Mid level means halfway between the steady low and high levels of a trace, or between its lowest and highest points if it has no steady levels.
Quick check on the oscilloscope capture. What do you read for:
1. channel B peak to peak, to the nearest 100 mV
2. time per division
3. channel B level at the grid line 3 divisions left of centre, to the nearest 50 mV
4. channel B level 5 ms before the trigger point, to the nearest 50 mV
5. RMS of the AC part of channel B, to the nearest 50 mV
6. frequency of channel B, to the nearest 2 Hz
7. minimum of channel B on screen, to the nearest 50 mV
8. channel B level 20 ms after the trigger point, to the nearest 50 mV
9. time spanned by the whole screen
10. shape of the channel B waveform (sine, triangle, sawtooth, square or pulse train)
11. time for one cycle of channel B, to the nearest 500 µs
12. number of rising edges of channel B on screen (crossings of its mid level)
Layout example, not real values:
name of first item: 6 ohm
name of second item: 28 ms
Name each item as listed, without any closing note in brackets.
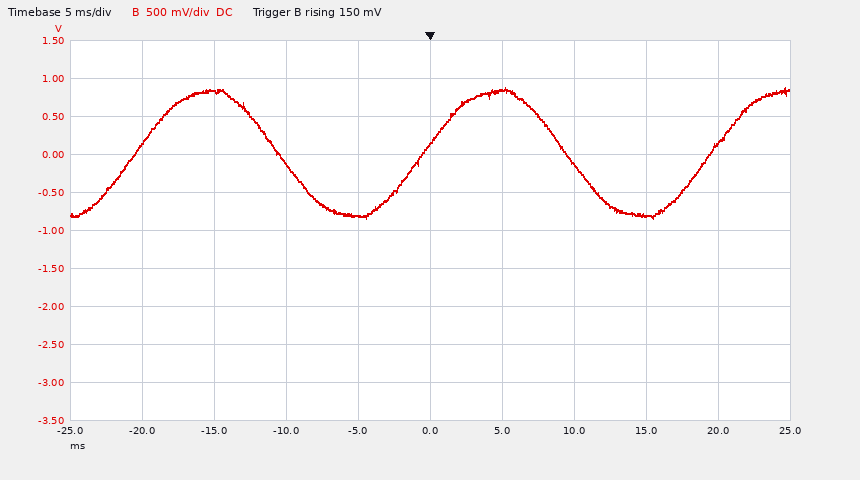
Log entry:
channel B peak to peak, to the nearest 100 mV: 1.70 V
time per division: 5 ms
channel B level at the grid line 3 divisions left of centre, to the nearest 50 mV: 800 mV
channel B level 5 ms before the trigger point, to the nearest 50 mV: -800 mV
RMS of the AC part of channel B, to the nearest 50 mV: 600 mV
frequency of channel B, to the nearest 2 Hz: 50 Hz
minimum of channel B on screen, to the nearest 50 mV: -850 mV
channel B level 20 ms after the trigger point, to the nearest 50 mV: 150 mV
time spanned by the whole screen: 50 ms
shape of the channel B waveform: sine
time for one cycle of channel B, to the nearest 500 µs: 20.0 ms
number of rising edges of channel B on screen: 3
